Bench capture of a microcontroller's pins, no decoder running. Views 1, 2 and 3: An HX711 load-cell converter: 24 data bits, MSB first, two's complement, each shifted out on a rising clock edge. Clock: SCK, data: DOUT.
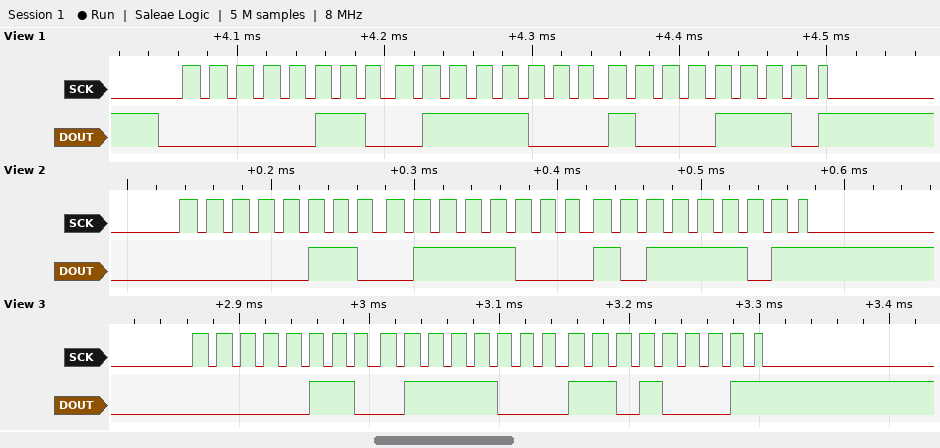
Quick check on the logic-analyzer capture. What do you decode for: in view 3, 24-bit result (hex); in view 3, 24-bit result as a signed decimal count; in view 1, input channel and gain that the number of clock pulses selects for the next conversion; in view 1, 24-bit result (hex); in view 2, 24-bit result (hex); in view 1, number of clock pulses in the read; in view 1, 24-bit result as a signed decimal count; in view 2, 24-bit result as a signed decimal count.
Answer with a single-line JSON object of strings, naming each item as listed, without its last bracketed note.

{"in view 3, 24-bit result": "0x0678D1", "in view 3, 24-bit result as a signed decimal count": "424145", "in view 1, input channel and gain that the number of clock pulses selects for the next conversion": "channel A, gain 128", "in view 1, 24-bit result": "0x06788E", "in view 2, 24-bit result": "0x0678BD", "in view 1, number of clock pulses in the read": "25", "in view 1, 24-bit result as a signed decimal count": "424078", "in view 2, 24-bit result as a signed decimal count": "424125"}
